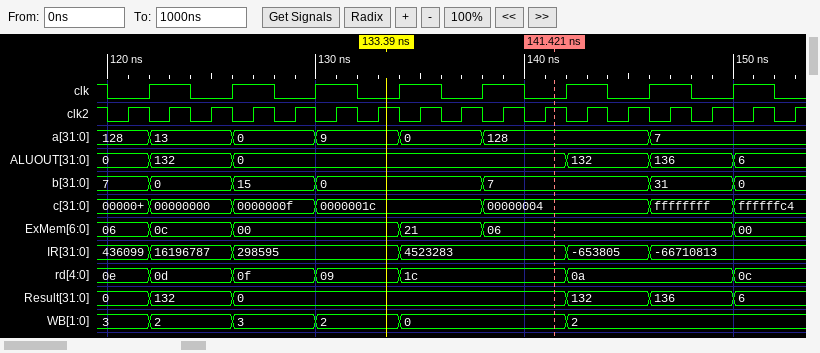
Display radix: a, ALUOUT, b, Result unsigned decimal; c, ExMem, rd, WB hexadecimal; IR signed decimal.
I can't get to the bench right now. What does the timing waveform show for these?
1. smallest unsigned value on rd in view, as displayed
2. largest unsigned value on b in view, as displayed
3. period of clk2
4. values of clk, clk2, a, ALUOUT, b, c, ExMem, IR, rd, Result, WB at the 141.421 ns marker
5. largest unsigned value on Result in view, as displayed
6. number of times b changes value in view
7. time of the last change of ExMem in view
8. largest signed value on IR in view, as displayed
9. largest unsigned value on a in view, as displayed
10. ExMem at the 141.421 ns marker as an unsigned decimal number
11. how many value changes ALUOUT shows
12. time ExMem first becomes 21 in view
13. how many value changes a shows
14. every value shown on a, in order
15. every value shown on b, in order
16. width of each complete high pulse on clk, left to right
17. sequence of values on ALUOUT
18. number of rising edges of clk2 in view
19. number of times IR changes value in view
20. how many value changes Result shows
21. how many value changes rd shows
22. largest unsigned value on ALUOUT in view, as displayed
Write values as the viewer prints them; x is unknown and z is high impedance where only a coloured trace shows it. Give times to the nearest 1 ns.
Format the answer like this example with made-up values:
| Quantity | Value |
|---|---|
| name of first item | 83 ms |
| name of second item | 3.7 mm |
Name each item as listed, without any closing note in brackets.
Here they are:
| Quantity | Value |
|---|---|
| smallest unsigned value on rd in view, as displayed | 09 |
| largest unsigned value on b in view, as displayed | 31 |
| period of clk2 | 2 ns |
| values of clk, clk2, a, ALUOUT, b, c, ExMem, IR, rd, Result, WB at the 141.421 ns marker | clk=0, clk2=1, a=128, ALUOUT=0, b=7, c=00000004, ExMem=06, IR=4523283, rd=1c, Result=0, WB=0 |
| largest unsigned value on Result in view, as displayed | 136 |
| number of times b changes value in view | 6 |
| time of the last change of ExMem in view | 150 ns |
| largest signed value on IR in view, as displayed | 16196787 |
| largest unsigned value on a in view, as displayed | 128 |
| ExMem at the 141.421 ns marker as an unsigned decimal number | 6 |
| how many value changes ALUOUT shows | 5 |
| time ExMem first becomes 21 in view | 134 ns |
| how many value changes a shows | 6 |
| every value shown on a, in order | 128, 13, 0, 9, 0, 128, 7 |
| every value shown on b, in order | 7, 0, 15, 0, 7, 31, 0 |
| width of each complete high pulse on clk, left to right | 2 ns, 2 ns, 2 ns, 2 ns, 2 ns, 2 ns, 2 ns, 2 ns |
| sequence of values on ALUOUT | 0, 132, 0, 132, 136, 6 |
| number of rising edges of clk2 in view | 17 |
| number of times IR changes value in view | 5 |
| how many value changes Result shows | 5 |
| how many value changes rd shows | 6 |
| largest unsigned value on ALUOUT in view, as displayed | 136 |
